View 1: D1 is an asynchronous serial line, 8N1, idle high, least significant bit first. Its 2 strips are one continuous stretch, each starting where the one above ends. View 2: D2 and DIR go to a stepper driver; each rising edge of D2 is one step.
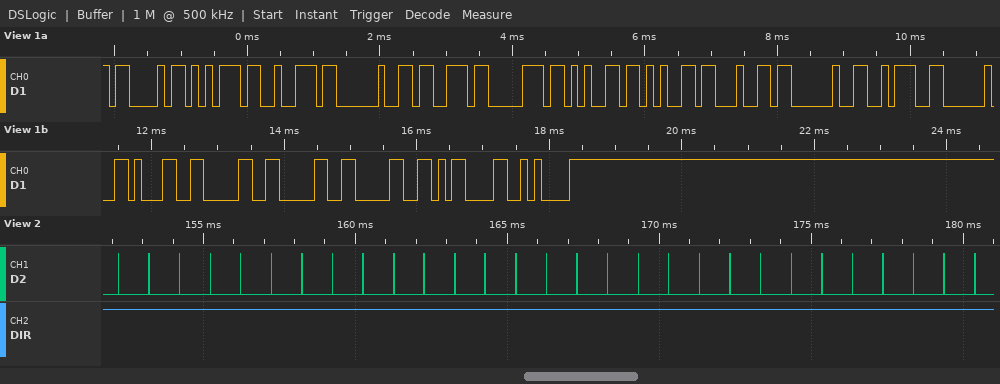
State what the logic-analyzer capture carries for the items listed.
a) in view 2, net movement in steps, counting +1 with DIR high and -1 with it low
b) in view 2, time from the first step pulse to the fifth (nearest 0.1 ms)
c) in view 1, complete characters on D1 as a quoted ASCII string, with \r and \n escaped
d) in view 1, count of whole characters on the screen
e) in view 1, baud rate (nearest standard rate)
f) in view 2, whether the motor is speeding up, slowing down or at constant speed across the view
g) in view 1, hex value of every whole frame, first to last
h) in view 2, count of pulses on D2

+29
4.0 ms
"Cur speed : 1000\r\n"
18
9600 baud
constant speed
0x43 0x75 0x72 0x20 0x73 0x70 0x65 0x65 0x64 0x20 0x3A 0x20 0x31 0x30 0x30 0x30 0x0D 0x0A
29
